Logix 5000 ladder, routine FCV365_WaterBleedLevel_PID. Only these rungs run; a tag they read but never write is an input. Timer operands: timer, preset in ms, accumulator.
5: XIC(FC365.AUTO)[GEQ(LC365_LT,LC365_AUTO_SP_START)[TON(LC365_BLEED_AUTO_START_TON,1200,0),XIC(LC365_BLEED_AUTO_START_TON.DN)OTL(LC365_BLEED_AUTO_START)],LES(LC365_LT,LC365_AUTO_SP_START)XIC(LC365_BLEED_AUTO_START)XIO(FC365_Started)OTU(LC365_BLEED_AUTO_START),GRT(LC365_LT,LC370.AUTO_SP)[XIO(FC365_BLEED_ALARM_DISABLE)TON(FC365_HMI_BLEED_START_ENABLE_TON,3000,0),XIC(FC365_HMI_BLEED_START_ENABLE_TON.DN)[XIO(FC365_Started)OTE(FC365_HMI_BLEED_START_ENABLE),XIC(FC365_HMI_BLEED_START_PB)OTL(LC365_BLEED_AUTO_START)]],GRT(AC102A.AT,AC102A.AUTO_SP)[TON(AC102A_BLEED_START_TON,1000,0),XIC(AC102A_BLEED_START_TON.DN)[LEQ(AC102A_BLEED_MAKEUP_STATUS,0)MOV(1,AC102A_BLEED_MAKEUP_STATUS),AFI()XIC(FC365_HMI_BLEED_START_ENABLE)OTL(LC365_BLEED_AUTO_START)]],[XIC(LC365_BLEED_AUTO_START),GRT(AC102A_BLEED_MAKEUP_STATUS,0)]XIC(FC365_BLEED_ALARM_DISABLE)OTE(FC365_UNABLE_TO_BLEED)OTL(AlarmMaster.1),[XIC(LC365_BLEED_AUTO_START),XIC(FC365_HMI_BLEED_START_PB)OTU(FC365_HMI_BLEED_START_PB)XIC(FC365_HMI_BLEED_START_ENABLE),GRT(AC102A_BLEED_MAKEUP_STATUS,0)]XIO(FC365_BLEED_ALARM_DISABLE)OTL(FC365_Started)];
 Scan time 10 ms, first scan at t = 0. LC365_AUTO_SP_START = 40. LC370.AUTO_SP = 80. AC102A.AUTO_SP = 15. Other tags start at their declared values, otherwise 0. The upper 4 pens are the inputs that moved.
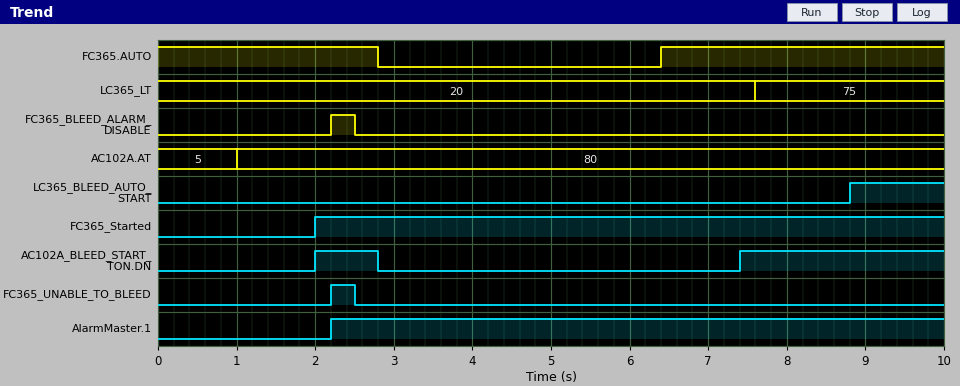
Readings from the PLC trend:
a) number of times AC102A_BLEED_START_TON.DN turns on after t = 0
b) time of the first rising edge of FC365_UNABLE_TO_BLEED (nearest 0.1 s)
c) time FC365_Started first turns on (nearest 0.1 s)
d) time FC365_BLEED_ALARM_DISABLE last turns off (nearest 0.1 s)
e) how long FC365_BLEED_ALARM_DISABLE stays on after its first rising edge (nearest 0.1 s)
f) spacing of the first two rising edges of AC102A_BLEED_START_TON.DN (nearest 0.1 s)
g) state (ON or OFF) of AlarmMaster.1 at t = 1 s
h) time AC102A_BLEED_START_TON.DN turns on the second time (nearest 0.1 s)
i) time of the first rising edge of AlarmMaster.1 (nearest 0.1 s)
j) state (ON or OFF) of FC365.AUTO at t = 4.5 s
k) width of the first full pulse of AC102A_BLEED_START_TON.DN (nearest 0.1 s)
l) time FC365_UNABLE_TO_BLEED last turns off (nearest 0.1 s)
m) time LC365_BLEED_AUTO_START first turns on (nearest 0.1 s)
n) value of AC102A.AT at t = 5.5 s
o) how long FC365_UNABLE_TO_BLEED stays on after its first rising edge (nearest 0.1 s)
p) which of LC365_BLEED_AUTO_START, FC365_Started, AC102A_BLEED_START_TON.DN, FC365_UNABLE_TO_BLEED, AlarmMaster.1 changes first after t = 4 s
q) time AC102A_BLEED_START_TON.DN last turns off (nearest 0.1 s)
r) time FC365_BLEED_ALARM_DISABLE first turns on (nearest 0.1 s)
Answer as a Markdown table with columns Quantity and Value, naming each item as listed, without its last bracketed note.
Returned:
| Quantity | Value |
|---|---|
| number of times AC102A_BLEED_START_TON.DN turns on after t = 0 | 2 |
| time of the first rising edge of FC365_UNABLE_TO_BLEED | 2.2 s |
| time FC365_Started first turns on | 2.0 s |
| time FC365_BLEED_ALARM_DISABLE last turns off | 2.5 s |
| how long FC365_BLEED_ALARM_DISABLE stays on after its first rising edge | 0.3 s |
| spacing of the first two rising edges of AC102A_BLEED_START_TON.DN | 5.4 s |
| state (ON or OFF) of AlarmMaster.1 at t = 1 s | OFF |
| time AC102A_BLEED_START_TON.DN turns on the second time | 7.4 s |
| time of the first rising edge of AlarmMaster.1 | 2.2 s |
| state (ON or OFF) of FC365.AUTO at t = 4.5 s | OFF |
| width of the first full pulse of AC102A_BLEED_START_TON.DN | 0.8 s |
| time FC365_UNABLE_TO_BLEED last turns off | 2.5 s |
| time LC365_BLEED_AUTO_START first turns on | 8.8 s |
| value of AC102A.AT at t = 5.5 s | 80 |
| how long FC365_UNABLE_TO_BLEED stays on after its first rising edge | 0.3 s |
| which of LC365_BLEED_AUTO_START, FC365_Started, AC102A_BLEED_START_TON.DN, FC365_UNABLE_TO_BLEED, AlarmMaster.1 changes first after t = 4 s | AC102A_BLEED_START_TON.DN |
| time AC102A_BLEED_START_TON.DN last turns off | 2.8 s |
| time FC365_BLEED_ALARM_DISABLE first turns on | 2.2 s |
